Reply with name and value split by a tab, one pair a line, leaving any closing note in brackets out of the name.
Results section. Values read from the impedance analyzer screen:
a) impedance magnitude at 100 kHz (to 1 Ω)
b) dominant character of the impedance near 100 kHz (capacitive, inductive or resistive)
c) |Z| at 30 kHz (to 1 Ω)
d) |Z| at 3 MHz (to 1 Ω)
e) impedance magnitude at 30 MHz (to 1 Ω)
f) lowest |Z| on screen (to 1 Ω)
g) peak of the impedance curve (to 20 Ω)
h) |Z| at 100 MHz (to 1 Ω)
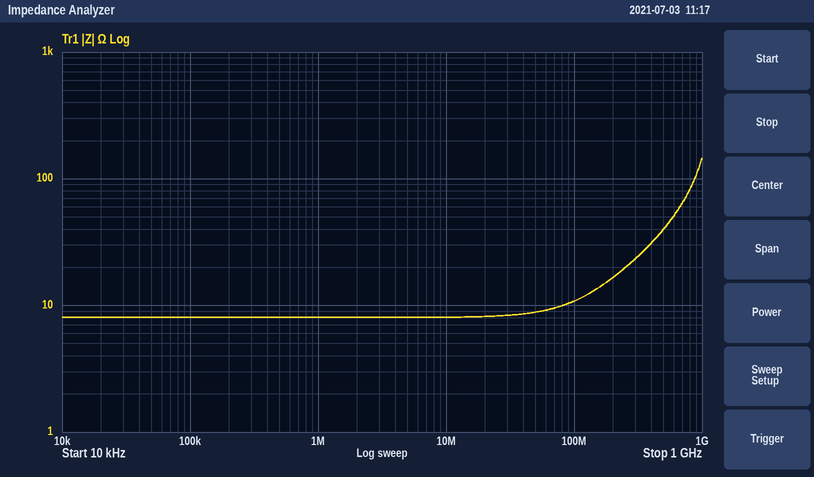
impedance magnitude at 100 kHz	8 Ω
dominant character of the impedance near 100 kHz	resistive
|Z| at 30 kHz	8 Ω
|Z| at 3 MHz	8 Ω
impedance magnitude at 30 MHz	8 Ω
lowest |Z| on screen	8 Ω
peak of the impedance curve	140 Ω
|Z| at 100 MHz	11 Ω
